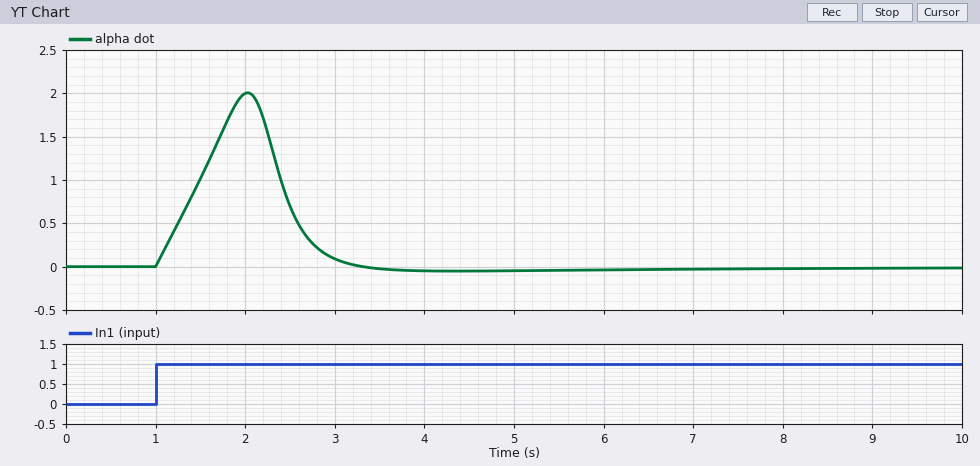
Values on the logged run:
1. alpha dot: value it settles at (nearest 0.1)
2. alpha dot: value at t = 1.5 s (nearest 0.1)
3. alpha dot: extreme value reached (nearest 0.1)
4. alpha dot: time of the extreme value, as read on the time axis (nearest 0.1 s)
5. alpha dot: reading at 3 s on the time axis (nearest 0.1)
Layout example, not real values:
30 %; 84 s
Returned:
0.0; 1.0; 2.0; 2.0 s; 0.1
